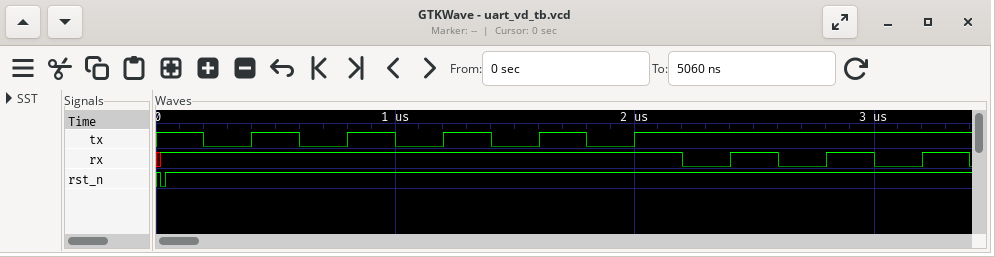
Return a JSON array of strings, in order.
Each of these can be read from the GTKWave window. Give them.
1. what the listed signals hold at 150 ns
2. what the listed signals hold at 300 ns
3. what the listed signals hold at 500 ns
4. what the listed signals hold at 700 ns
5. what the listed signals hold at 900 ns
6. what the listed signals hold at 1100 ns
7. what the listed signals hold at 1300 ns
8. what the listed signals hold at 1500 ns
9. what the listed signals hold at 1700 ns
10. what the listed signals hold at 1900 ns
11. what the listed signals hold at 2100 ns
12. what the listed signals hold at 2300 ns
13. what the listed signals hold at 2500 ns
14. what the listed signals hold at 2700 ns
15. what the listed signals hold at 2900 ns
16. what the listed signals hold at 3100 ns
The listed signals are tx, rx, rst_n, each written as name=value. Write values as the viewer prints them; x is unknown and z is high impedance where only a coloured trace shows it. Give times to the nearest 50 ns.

["tx=1, rx=1, rst_n=1", "tx=0, rx=1, rst_n=1", "tx=1, rx=1, rst_n=1", "tx=0, rx=1, rst_n=1", "tx=1, rx=1, rst_n=1", "tx=0, rx=1, rst_n=1", "tx=1, rx=1, rst_n=1", "tx=0, rx=1, rst_n=1", "tx=1, rx=1, rst_n=1", "tx=0, rx=1, rst_n=1", "tx=1, rx=1, rst_n=1", "tx=1, rx=0, rst_n=1", "tx=1, rx=1, rst_n=1", "tx=1, rx=0, rst_n=1", "tx=1, rx=1, rst_n=1", "tx=1, rx=0, rst_n=1"]
